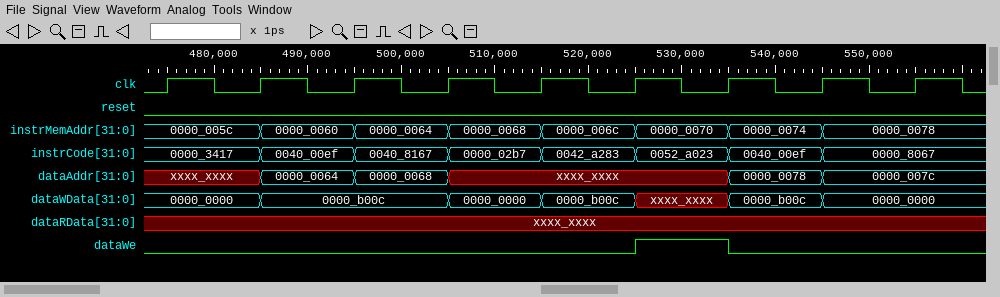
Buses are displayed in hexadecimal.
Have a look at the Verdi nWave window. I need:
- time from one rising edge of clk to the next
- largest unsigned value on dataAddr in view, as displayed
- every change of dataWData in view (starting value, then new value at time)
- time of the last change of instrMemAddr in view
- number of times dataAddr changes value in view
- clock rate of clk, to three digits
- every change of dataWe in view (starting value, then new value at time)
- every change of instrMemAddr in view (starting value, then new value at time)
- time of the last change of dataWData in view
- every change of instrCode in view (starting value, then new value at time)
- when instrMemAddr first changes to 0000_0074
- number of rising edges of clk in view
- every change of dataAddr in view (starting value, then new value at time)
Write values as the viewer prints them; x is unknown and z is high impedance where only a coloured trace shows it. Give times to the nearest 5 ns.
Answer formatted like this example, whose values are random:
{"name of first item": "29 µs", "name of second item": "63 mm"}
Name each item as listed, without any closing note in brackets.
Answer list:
{"time from one rising edge of clk to the next": "10 ns", "largest unsigned value on dataAddr in view, as displayed": "0000_007c", "every change of dataWData in view": "0000_0000, 0000_b00c at 485 ns, 0000_0000 at 505 ns, 0000_b00c at 515 ns, xxxx_xxxx at 525 ns, 0000_b00c at 535 ns, 0000_0000 at 545 ns", "time of the last change of instrMemAddr in view": "545 ns", "number of times dataAddr changes value in view": "5", "clock rate of clk, to three digits": "100 MHz", "every change of dataWe in view": "0, 1 at 525 ns, 0 at 535 ns", "every change of instrMemAddr in view": "0000_005c, 0000_0060 at 485 ns, 0000_0064 at 495 ns, 0000_0068 at 505 ns, 0000_006c at 515 ns, 0000_0070 at 525 ns, 0000_0074 at 535 ns, 0000_0078 at 545 ns", "time of the last change of dataWData in view": "545 ns", "every change of instrCode in view": "0000_3417, 0040_00ef at 485 ns, 0040_8167 at 495 ns, 0000_02b7 at 505 ns, 0042_a283 at 515 ns, 0052_a023 at 525 ns, 0040_00ef at 535 ns, 0000_8067 at 545 ns", "when instrMemAddr first changes to 0000_0074": "535 ns", "number of rising edges of clk in view": "9", "every change of dataAddr in view": "xxxx_xxxx, 0000_0064 at 485 ns, 0000_0068 at 495 ns, xxxx_xxxx at 505 ns, 0000_0078 at 535 ns, 0000_007c at 545 ns"}
